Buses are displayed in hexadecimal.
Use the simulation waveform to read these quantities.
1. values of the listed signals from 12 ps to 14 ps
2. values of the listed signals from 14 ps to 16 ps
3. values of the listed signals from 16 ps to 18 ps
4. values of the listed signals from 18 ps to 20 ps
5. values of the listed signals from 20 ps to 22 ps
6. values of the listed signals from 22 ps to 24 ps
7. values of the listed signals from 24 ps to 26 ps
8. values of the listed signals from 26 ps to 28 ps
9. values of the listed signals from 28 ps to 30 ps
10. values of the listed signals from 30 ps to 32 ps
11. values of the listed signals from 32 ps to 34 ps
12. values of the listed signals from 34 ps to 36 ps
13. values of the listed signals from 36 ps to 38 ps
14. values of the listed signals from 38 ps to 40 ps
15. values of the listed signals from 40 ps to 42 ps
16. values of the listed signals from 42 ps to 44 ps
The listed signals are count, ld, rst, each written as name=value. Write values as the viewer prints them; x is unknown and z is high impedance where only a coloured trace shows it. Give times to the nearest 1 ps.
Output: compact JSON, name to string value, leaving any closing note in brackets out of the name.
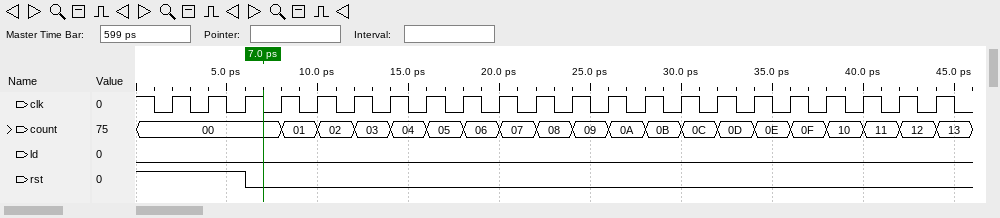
{"values of the listed signals from 12 ps to 14 ps": "count=03, ld=0, rst=0", "values of the listed signals from 14 ps to 16 ps": "count=04, ld=0, rst=0", "values of the listed signals from 16 ps to 18 ps": "count=05, ld=0, rst=0", "values of the listed signals from 18 ps to 20 ps": "count=06, ld=0, rst=0", "values of the listed signals from 20 ps to 22 ps": "count=07, ld=0, rst=0", "values of the listed signals from 22 ps to 24 ps": "count=08, ld=0, rst=0", "values of the listed signals from 24 ps to 26 ps": "count=09, ld=0, rst=0", "values of the listed signals from 26 ps to 28 ps": "count=0A, ld=0, rst=0", "values of the listed signals from 28 ps to 30 ps": "count=0B, ld=0, rst=0", "values of the listed signals from 30 ps to 32 ps": "count=0C, ld=0, rst=0", "values of the listed signals from 32 ps to 34 ps": "count=0D, ld=0, rst=0", "values of the listed signals from 34 ps to 36 ps": "count=0E, ld=0, rst=0", "values of the listed signals from 36 ps to 38 ps": "count=0F, ld=0, rst=0", "values of the listed signals from 38 ps to 40 ps": "count=10, ld=0, rst=0", "values of the listed signals from 40 ps to 42 ps": "count=11, ld=0, rst=0", "values of the listed signals from 42 ps to 44 ps": "count=12, ld=0, rst=0"}
